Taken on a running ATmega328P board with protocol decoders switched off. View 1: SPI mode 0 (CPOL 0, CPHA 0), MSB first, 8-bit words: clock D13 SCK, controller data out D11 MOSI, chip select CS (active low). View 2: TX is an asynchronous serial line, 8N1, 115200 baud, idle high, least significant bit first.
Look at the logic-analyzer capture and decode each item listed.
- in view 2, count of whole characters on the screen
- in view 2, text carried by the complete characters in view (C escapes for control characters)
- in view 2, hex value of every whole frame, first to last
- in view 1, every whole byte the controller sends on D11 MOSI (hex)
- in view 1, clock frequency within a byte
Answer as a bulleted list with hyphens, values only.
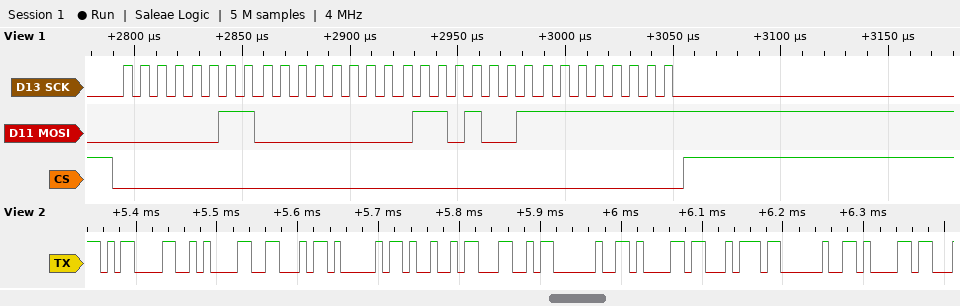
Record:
- 11
- "\r\nFAIL at a"
- 0D 0A 46 41 49 4C 20 61 74 20 61
- 03 00 69 FF
- 125 kHz
